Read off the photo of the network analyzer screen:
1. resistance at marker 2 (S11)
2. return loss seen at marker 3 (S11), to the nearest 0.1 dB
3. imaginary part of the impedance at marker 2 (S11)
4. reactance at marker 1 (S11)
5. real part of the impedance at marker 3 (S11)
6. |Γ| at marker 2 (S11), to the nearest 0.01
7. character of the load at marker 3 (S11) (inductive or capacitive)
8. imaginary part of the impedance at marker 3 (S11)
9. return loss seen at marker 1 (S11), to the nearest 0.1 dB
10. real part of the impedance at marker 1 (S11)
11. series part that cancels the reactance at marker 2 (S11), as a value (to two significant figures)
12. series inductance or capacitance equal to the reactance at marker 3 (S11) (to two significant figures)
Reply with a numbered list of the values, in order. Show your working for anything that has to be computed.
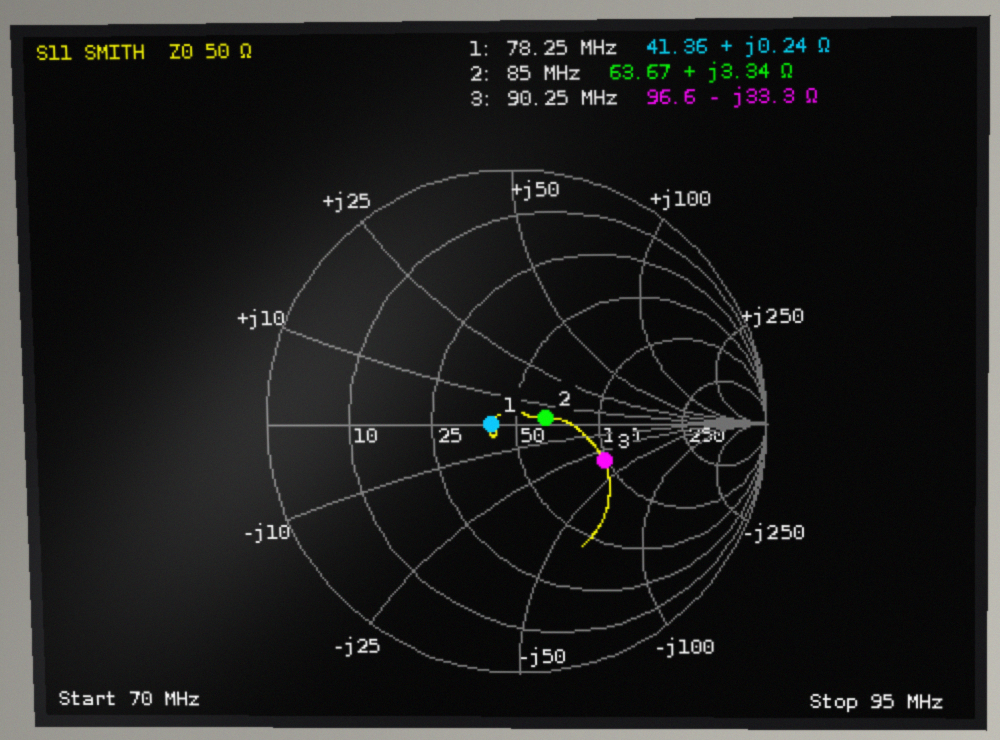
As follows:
1. 63.67 Ω
2. 8.4 dB
3. +3.34 Ω
4. +0.24 Ω
5. 96.6 Ω
6. 0.12
7. capacitive
8. -33.3 Ω
9. 20.5 dB
10. 41.36 Ω
11. C = 1/(2π × 85 MHz × 3.34 Ω) ≈ 561 pF, so 560 pF to two significant figures
12. C = 1/(2π × 90.25 MHz × 33.3 Ω) ≈ 53 pF
